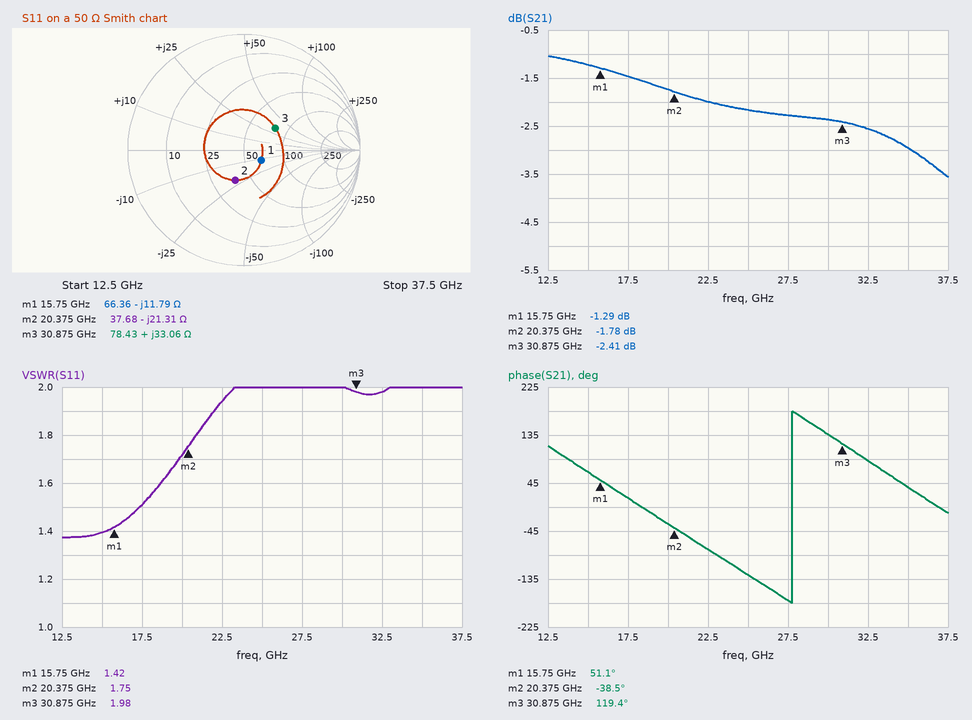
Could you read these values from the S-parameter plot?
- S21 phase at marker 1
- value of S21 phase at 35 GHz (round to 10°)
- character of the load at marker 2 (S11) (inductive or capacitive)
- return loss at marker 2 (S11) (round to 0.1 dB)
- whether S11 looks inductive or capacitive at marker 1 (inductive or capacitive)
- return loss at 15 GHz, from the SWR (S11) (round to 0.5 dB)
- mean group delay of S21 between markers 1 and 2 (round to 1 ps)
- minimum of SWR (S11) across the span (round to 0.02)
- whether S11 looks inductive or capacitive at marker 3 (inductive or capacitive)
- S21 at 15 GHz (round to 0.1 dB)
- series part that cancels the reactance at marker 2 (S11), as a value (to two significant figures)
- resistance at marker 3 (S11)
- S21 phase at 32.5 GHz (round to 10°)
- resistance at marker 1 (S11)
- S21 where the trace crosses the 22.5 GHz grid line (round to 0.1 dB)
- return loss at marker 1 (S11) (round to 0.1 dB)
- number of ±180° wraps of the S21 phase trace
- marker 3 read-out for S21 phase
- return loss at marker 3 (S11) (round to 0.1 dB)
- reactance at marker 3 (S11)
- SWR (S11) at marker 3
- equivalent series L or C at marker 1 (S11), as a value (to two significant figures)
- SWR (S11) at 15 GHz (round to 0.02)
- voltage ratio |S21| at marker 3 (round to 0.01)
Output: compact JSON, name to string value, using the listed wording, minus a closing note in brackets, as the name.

{"S21 phase at marker 1": "51.1°", "value of S21 phase at 35 GHz": "40°", "character of the load at marker 2 (S11)": "capacitive", "return loss at marker 2 (S11)": "11.3 dB", "whether S11 looks inductive or capacitive at marker 1": "capacitive", "return loss at 15 GHz, from the SWR (S11)": "15.5 dB", "mean group delay of S21 between markers 1 and 2": "54 ps", "minimum of SWR (S11) across the span": "1.38", "whether S11 looks inductive or capacitive at marker 3": "inductive", "S21 at 15 GHz": "-1.2 dB", "series part that cancels the reactance at marker 2 (S11), as a value": "170 pH", "resistance at marker 3": "78.43 Ω", "S21 phase at 32.5 GHz": "90°", "resistance at marker 1": "66.36 Ω", "S21 where the trace crosses the 22.5 GHz grid line": "-2.0 dB", "return loss at marker 1 (S11)": "15.3 dB", "number of ±180° wraps of the S21 phase trace": "1", "marker 3 read-out for S21 phase": "119.4°", "return loss at marker 3 (S11)": "9.7 dB", "reactance at marker 3": "+33.06 Ω", "SWR (S11) at marker 3": "1.98", "equivalent series L or C at marker 1 (S11), as a value": "860 fF", "SWR (S11) at 15 GHz": "1.40", "voltage ratio |S21| at marker 3": "0.76"}
